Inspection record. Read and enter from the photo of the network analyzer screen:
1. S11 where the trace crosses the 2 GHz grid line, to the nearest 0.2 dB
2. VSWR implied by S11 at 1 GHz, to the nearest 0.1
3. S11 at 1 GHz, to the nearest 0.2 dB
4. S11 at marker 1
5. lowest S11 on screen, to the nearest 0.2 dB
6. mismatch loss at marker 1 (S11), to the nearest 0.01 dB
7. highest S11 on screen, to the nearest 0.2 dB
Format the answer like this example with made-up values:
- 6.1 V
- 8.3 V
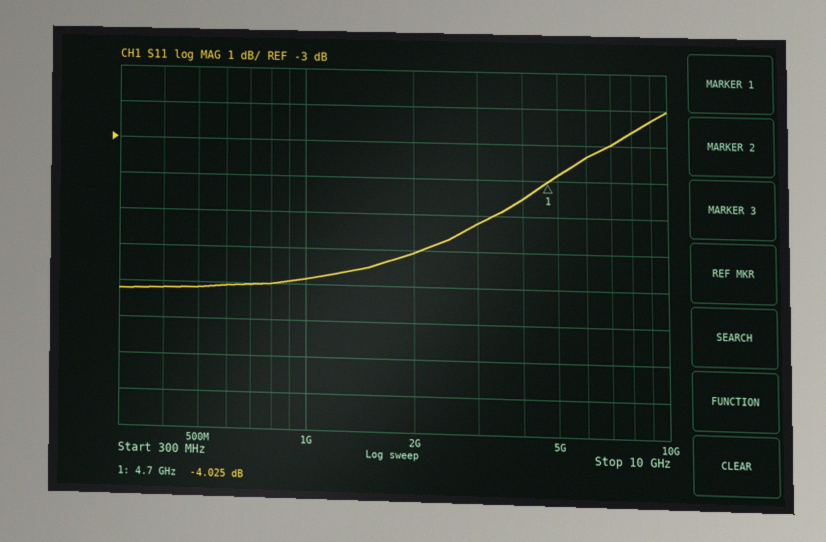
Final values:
- -6.0 dB
- 2.7
- -6.8 dB
- -4.025 dB
- -7.2 dB
- 2.19 dB
- -2.0 dB
